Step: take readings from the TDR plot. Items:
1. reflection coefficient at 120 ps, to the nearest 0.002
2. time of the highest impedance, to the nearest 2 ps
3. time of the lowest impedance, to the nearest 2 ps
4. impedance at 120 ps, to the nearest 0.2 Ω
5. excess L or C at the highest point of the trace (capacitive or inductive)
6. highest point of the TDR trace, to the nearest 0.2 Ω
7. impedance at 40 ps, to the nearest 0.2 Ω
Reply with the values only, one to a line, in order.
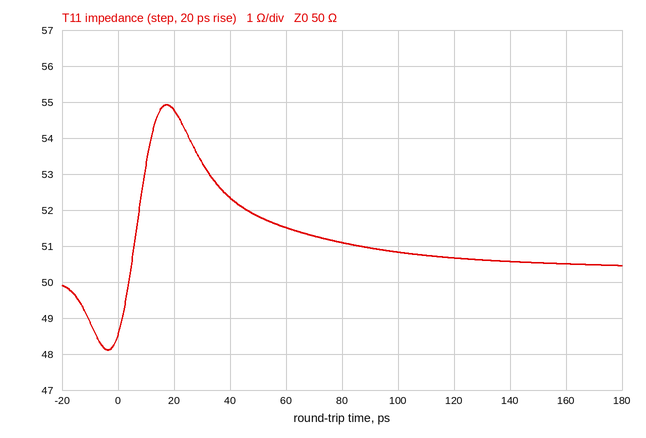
+0.006
18 ps
-4 ps
50.6 Ω
inductive
55.0 Ω
52.4 Ω
